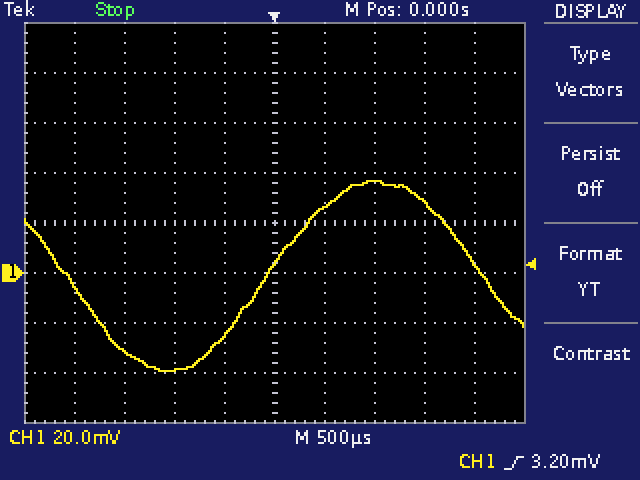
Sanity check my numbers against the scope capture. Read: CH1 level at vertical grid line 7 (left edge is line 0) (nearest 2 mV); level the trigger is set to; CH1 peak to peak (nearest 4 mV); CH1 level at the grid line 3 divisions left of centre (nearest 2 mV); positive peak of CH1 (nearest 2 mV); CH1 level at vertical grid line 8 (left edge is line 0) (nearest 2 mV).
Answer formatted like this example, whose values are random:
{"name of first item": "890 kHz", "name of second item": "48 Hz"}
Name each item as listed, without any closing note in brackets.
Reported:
{"CH1 level at vertical grid line 7 (left edge is line 0)": "36 mV", "level the trigger is set to": "3.20 mV", "CH1 peak to peak": "76 mV", "CH1 level at the grid line 3 divisions left of centre": "-32 mV", "positive peak of CH1": "36 mV", "CH1 level at vertical grid line 8 (left edge is line 0)": "28 mV"}
